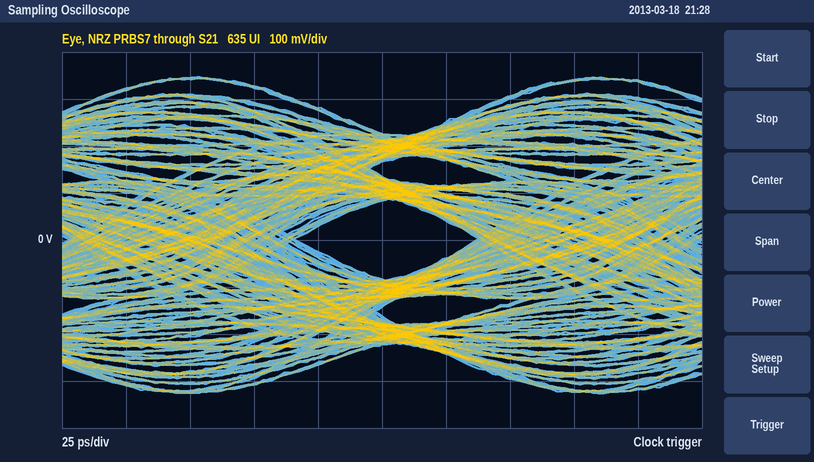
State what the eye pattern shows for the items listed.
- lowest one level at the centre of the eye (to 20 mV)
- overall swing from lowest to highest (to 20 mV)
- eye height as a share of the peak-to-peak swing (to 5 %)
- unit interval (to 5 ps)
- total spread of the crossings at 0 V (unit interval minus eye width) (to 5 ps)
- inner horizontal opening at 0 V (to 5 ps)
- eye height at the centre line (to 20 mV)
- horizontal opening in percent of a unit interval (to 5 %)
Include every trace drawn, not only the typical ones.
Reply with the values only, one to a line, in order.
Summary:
80 mV
680 mV
25 %
160 ps
90 ps
70 ps
160 mV
45 %
